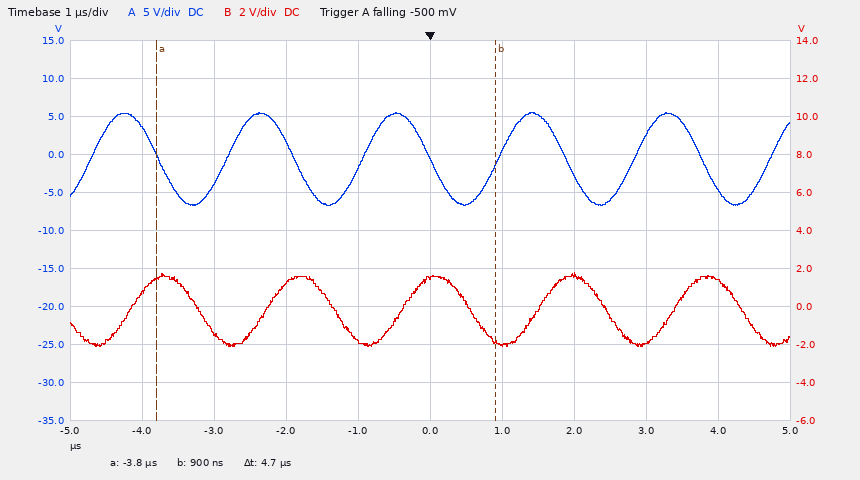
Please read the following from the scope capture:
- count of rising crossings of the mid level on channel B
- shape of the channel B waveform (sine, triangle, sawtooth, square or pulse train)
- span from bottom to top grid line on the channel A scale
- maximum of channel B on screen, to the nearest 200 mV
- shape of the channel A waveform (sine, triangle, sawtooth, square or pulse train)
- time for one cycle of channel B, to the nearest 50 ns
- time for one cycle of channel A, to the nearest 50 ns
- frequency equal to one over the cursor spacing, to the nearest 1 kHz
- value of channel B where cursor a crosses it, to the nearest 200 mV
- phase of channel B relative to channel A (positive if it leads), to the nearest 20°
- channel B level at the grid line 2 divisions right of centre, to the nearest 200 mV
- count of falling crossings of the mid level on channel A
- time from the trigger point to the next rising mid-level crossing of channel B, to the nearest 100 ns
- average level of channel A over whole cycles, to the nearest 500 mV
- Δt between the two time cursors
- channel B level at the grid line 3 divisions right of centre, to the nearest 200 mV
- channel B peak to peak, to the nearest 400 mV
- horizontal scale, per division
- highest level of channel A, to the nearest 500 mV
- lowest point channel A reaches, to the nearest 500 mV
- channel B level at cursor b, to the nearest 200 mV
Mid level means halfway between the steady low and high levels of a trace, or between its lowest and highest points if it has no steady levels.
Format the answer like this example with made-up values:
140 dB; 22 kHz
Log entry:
5; sine; 50 V; 1.8 V; sine; 1.90 µs; 1.90 µs; 213 kHz; 1.4 V; -100°; 1.6 V; 5; 1.5 µs; -500 mV; 4.7 µs; -2.0 V; 4.0 V; 1 µs; 5.5 V; -6.5 V; -1.8 V
